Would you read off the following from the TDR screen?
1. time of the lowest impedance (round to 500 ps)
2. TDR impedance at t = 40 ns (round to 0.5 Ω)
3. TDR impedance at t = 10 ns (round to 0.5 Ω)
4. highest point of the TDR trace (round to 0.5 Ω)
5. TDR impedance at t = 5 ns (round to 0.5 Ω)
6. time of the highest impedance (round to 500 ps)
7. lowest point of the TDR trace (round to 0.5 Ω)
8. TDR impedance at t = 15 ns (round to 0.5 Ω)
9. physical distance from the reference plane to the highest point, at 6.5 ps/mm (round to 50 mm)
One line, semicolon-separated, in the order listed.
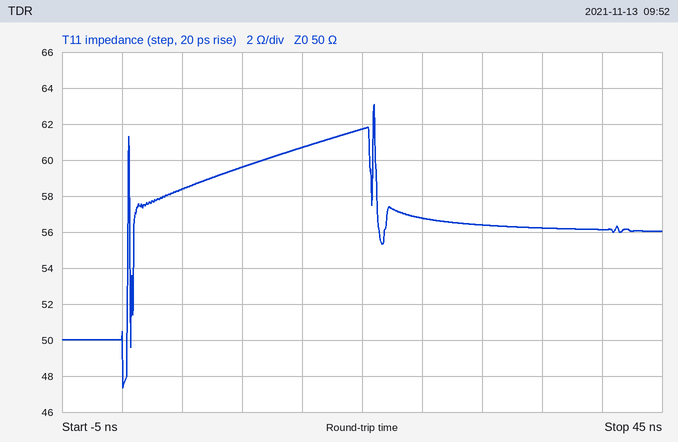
0.0 ns; 56.0 Ω; 59.5 Ω; 63.0 Ω; 58.5 Ω; 21.0 ns; 47.5 Ω; 60.5 Ω; 1.60 m
